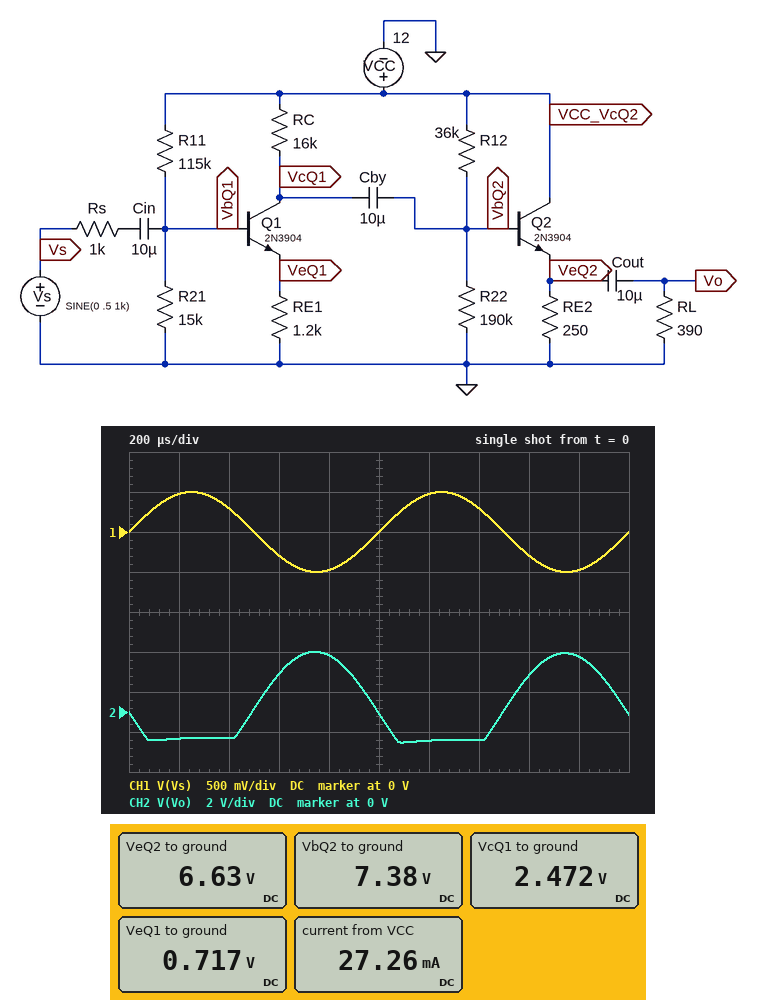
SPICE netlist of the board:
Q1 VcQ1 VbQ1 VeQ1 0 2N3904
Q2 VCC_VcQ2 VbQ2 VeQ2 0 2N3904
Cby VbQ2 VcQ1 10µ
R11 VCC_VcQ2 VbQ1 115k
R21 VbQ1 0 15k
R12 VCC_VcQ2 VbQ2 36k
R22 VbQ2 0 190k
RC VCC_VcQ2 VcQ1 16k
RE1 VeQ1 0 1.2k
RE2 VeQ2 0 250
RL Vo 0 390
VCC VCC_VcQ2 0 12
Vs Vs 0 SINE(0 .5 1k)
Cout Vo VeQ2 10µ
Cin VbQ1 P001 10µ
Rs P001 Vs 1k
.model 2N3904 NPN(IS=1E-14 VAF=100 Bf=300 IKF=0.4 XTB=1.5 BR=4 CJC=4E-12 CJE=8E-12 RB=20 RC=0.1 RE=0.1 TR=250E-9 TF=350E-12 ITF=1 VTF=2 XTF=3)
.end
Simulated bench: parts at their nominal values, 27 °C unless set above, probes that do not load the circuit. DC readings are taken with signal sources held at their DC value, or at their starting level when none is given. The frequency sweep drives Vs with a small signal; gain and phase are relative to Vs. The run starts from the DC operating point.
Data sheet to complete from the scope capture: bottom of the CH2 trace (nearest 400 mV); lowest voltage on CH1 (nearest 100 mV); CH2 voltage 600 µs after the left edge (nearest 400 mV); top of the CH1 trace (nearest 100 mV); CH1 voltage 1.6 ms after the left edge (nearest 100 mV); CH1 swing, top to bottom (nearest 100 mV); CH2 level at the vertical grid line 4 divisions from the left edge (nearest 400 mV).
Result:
-1.6 V
-500 mV
2.0 V
500 mV
-300 mV
1.0 V
2.8 V
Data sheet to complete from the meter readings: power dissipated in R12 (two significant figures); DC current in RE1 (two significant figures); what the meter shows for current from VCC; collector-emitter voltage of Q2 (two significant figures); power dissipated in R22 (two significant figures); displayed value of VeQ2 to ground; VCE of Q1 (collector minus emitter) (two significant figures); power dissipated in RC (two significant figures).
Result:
590 µW
600 µA
27.26 mA
5.4 V
290 µW
6.63 V
1.8 V
5.7 mW
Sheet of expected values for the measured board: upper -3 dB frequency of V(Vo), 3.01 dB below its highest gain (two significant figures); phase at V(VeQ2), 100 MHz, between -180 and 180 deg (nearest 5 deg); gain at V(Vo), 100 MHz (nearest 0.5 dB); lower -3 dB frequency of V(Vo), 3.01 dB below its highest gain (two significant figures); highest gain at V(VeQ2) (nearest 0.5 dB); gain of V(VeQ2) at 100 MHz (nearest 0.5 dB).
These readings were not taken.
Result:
1.9 MHz
-20 deg
-13.0 dB
38 Hz
16.5 dB
-13.0 dB
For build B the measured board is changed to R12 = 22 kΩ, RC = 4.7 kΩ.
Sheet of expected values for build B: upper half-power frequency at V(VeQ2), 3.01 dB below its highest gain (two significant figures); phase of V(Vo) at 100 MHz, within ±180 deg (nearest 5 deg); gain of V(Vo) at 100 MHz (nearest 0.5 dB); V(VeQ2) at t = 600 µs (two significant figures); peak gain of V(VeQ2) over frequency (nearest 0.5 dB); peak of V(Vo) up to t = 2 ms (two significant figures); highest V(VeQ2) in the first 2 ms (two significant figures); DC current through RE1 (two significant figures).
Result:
5.4 MHz
-5 deg
-13.5 dB
8.6 V
8.5 dB
1.3 V
9.1 V
600 µA
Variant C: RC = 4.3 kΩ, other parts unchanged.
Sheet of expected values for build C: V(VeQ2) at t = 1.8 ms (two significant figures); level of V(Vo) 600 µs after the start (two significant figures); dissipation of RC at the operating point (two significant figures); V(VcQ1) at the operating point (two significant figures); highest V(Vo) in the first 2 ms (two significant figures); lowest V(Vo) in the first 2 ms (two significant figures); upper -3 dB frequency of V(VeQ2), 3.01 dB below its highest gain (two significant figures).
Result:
7.8 V
830 mV
1.5 mW
9.4 V
1.3 V
-1.2 V
5.6 MHz
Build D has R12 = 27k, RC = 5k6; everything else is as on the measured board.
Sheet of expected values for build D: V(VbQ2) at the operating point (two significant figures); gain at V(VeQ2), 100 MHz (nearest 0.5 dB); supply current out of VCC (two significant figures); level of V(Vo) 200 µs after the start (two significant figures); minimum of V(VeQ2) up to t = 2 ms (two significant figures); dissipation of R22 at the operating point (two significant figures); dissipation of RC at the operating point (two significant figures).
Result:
8.1 V
-13.5 dB
30 mA
-1.4 V
5.9 V
350 µW
2.0 mW
